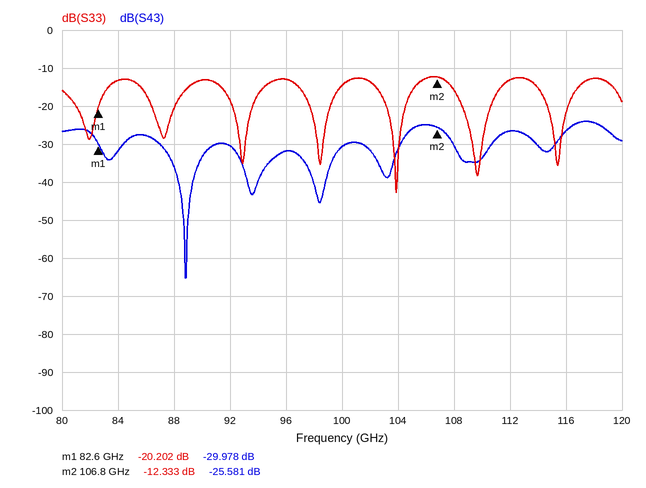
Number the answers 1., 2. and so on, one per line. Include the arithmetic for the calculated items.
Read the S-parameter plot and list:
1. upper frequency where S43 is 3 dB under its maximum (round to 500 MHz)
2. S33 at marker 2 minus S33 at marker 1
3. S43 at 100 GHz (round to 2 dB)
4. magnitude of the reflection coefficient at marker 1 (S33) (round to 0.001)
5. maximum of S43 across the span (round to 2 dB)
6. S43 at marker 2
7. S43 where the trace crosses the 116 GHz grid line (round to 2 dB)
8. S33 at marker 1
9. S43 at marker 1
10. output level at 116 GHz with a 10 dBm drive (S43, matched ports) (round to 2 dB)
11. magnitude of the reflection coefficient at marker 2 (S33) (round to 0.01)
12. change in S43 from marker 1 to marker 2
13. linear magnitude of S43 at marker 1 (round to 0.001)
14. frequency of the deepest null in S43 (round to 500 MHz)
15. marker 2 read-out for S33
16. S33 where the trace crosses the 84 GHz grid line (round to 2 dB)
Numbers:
1. 119.0 GHz
2. -12.333 − (-20.202) = 7.869 dB
3. -30 dB
4. 10^(-20.202/20) ≈ 0.098
5. -24 dB
6. -25.581 dB
7. -26 dB
8. -20.202 dB
9. -29.978 dB
10. 10 dBm + (-26 dB) = -16 dBm
11. 10^(-12.333/20) ≈ 0.24
12. -25.581 − (-29.978) = 4.397 dB
13. 10^(-29.978/20) ≈ 0.032
14. 89.0 GHz
15. -12.333 dB
16. -14 dB
